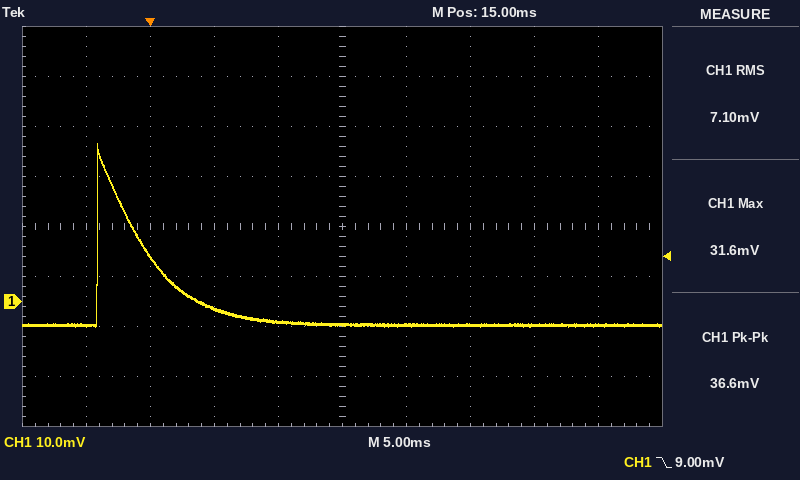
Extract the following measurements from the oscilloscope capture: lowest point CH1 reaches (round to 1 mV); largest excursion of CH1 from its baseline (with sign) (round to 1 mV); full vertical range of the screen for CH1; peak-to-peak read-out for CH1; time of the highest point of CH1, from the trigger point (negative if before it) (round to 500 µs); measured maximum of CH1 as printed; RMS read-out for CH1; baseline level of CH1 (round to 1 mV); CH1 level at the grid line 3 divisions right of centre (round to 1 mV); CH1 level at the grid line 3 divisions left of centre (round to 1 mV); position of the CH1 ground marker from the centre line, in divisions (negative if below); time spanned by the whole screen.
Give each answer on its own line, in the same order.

-5 mV
+36 mV
80 mV
36.6 mV
-4.0 ms
31.6 mV
7.10 mV
-5 mV
-5 mV
9 mV
-1.5 div
50 ms
